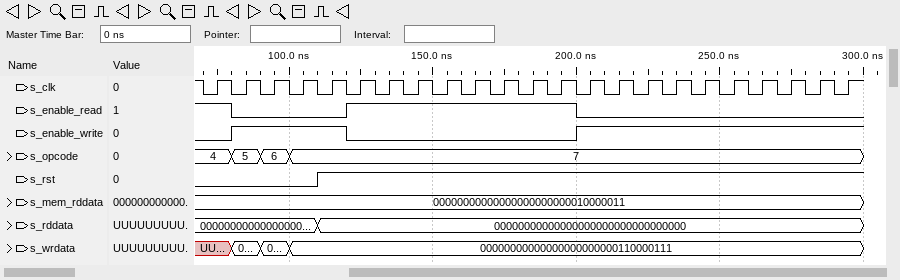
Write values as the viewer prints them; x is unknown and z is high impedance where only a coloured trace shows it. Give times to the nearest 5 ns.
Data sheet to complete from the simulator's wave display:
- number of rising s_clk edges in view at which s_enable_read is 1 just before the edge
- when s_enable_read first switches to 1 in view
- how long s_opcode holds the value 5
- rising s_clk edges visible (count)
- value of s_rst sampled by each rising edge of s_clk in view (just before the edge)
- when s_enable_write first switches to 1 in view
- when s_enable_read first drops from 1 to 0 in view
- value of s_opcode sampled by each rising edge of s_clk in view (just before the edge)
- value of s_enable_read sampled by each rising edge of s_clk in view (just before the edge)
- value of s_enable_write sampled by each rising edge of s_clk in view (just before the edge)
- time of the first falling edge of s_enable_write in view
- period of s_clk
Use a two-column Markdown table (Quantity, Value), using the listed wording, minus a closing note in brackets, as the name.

| Quantity | Value |
|---|---|
| number of rising s_clk edges in view at which s_enable_read is 1 just before the edge | 9 |
| when s_enable_read first switches to 1 in view | 120 ns |
| how long s_opcode holds the value 5 | 10 ns |
| rising s_clk edges visible | 23 |
| value of s_rst sampled by each rising edge of s_clk in view | 0 0 0 0 1 1 1 1 1 1 1 1 1 1 1 1 1 1 1 1 1 1 1 |
| when s_enable_write first switches to 1 in view | 80 ns |
| when s_enable_read first drops from 1 to 0 in view | 80 ns |
| value of s_opcode sampled by each rising edge of s_clk in view | 4, 5, 6, 7, 7, 7, 7, 7, 7, 7, 7, 7, 7, 7, 7, 7, 7, 7, 7, 7, 7, 7, 7 |
| value of s_enable_read sampled by each rising edge of s_clk in view | 1 0 0 0 0 1 1 1 1 1 1 1 1 0 0 0 0 0 0 0 0 0 0 |
| value of s_enable_write sampled by each rising edge of s_clk in view | 0 1 1 1 1 0 0 0 0 0 0 0 0 1 1 1 1 1 1 1 1 1 1 |
| time of the first falling edge of s_enable_write in view | 120 ns |
| period of s_clk | 10 ns |
